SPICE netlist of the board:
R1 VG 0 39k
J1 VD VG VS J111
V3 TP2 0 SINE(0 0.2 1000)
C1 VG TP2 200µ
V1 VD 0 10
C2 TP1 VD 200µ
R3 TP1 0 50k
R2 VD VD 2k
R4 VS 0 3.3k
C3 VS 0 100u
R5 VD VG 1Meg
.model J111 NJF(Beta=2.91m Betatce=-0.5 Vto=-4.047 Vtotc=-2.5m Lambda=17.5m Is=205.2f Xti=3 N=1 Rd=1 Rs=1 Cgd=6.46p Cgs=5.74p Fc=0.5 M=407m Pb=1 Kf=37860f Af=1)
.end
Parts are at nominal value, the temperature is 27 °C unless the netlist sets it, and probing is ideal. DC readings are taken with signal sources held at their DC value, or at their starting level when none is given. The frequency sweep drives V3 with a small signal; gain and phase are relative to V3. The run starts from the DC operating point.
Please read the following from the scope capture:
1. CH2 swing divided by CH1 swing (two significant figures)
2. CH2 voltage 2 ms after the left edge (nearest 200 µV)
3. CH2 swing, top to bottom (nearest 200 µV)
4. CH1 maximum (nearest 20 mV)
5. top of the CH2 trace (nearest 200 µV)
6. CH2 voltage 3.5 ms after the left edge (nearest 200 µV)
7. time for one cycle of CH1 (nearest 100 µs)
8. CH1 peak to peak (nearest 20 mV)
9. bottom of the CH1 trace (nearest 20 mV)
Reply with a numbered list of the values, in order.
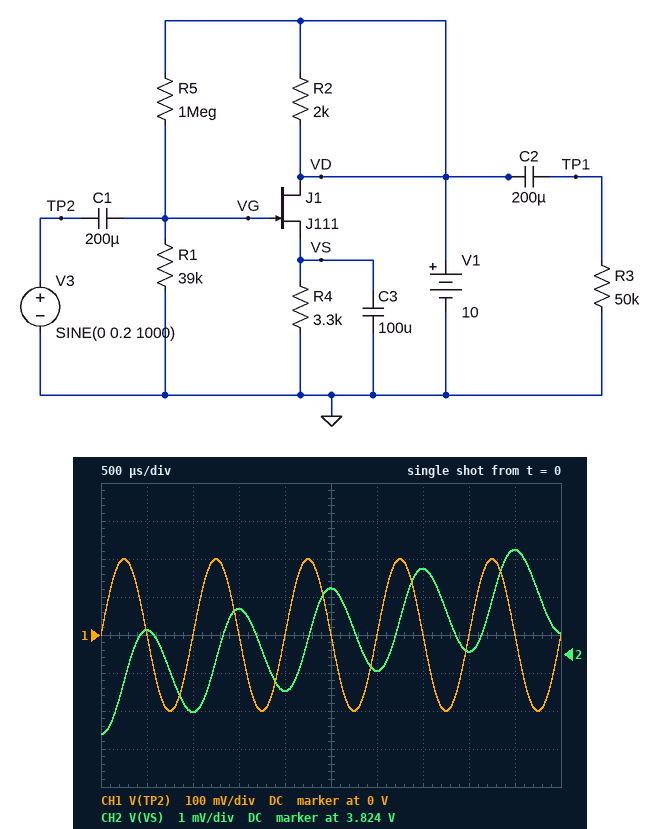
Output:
1. 0.012
2. 3.8230 V
3. 4.8 mV
4. 200 mV
5. 3.8268 V
6. 3.8262 V
7. 1.0 ms
8. 400 mV
9. -200 mV
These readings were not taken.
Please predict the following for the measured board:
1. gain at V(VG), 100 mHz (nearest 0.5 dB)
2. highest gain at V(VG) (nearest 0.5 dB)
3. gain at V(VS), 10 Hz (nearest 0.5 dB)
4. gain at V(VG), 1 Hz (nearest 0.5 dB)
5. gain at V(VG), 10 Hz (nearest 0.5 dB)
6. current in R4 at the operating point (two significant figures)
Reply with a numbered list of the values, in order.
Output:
1. 0 dB
2. 0 dB
3. -6.0 dB
4. 0 dB
5. 0 dB
6. 1.2 mA
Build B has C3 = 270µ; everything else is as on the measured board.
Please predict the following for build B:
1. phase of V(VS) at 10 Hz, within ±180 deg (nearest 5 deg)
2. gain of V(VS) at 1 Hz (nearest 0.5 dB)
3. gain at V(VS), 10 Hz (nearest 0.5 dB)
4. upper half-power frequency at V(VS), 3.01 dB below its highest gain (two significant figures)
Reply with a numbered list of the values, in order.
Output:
1. -75 deg
2. -1.5 dB
3. -13.0 dB
4. 2.5 Hz
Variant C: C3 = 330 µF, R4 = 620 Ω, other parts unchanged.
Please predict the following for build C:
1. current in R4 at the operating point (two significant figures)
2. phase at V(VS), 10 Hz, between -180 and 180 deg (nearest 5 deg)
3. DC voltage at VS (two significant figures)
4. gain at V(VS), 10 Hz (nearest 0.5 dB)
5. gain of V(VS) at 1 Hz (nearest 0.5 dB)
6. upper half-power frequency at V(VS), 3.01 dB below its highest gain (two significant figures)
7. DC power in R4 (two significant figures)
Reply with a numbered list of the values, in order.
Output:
1. 5.1 mA
2. -65 deg
3. 3.2 V
4. -9.0 dB
5. -2.0 dB
6. 4.8 Hz
7. 16 mW
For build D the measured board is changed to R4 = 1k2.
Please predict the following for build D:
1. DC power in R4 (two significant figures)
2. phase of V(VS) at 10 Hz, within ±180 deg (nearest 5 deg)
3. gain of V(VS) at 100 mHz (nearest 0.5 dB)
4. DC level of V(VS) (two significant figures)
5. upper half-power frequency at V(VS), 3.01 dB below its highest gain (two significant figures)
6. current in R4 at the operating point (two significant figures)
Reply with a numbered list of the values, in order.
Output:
1. 10 mW
2. -40 deg
3. -1.5 dB
4. 3.5 V
5. 11 Hz
6. 2.9 mA
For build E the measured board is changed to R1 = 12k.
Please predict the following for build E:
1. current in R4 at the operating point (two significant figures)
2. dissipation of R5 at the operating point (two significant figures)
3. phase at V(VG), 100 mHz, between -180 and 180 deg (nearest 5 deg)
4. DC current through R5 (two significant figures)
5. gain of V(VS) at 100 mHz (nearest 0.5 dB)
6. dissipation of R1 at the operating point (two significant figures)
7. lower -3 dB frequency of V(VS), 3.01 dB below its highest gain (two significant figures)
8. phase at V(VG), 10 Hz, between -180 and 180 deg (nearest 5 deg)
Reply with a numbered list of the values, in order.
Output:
1. 1.1 mA
2. 98 µW
3. 35 deg
4. 9.9 µA
5. -2.5 dB
6. 1.2 µW
7. 66 mHz
8. 0 deg
